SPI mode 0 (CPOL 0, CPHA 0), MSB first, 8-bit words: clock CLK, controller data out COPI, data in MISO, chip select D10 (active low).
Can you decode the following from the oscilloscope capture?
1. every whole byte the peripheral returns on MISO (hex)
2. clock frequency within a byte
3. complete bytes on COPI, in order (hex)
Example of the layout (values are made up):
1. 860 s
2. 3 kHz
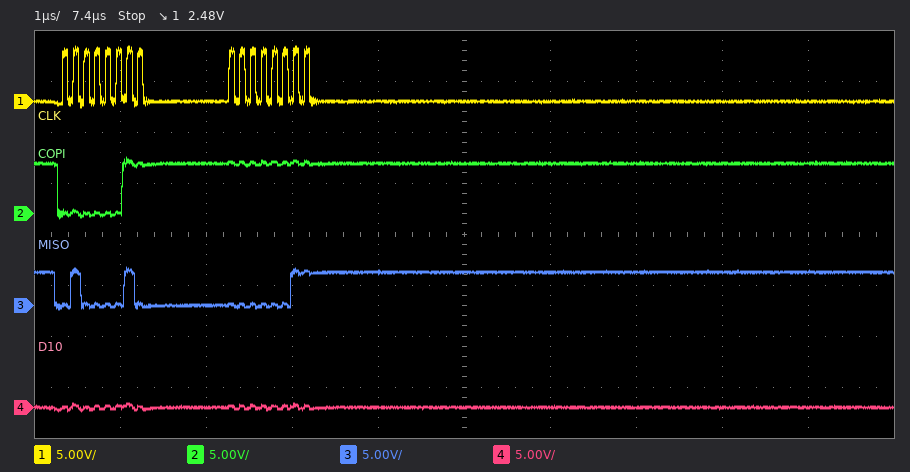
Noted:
1. 42 03
2. 8 MHz
3. 03 FF
